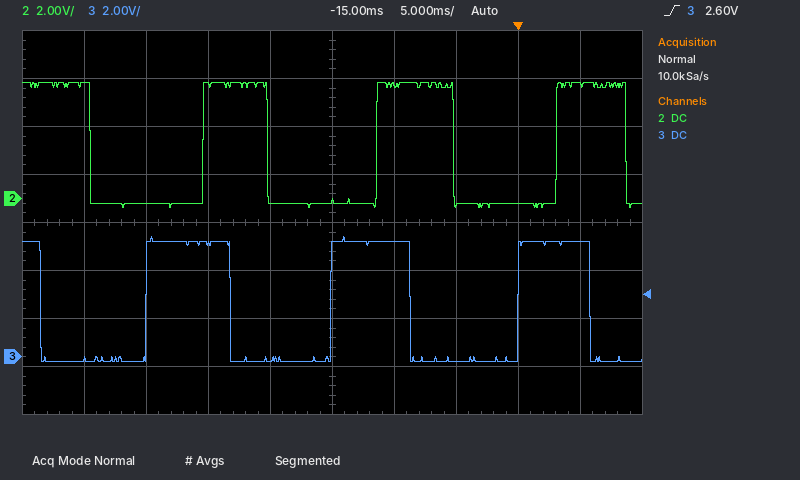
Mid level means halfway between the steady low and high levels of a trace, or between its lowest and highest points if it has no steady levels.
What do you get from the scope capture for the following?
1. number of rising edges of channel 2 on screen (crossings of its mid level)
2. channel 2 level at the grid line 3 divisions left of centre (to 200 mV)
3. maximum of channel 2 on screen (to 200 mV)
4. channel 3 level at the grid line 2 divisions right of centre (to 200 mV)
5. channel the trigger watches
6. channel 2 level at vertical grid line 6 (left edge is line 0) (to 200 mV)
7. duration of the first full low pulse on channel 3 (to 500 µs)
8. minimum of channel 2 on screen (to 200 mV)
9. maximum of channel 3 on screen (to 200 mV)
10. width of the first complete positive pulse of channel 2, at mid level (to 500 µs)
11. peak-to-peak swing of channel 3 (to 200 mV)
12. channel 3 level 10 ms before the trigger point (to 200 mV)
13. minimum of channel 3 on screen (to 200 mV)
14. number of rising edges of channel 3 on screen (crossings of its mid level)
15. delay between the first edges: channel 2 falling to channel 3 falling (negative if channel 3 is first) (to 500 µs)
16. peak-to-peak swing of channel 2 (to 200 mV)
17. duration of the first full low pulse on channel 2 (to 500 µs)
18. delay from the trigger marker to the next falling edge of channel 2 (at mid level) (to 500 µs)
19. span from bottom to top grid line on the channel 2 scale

3
-200 mV
4.8 V
-200 mV
channel 3
4.8 V
8.5 ms
-400 mV
5.0 V
5.0 ms
5.2 V
4.8 V
-200 mV
3
-4.0 ms
5.2 V
9.0 ms
8.5 ms
16 V
